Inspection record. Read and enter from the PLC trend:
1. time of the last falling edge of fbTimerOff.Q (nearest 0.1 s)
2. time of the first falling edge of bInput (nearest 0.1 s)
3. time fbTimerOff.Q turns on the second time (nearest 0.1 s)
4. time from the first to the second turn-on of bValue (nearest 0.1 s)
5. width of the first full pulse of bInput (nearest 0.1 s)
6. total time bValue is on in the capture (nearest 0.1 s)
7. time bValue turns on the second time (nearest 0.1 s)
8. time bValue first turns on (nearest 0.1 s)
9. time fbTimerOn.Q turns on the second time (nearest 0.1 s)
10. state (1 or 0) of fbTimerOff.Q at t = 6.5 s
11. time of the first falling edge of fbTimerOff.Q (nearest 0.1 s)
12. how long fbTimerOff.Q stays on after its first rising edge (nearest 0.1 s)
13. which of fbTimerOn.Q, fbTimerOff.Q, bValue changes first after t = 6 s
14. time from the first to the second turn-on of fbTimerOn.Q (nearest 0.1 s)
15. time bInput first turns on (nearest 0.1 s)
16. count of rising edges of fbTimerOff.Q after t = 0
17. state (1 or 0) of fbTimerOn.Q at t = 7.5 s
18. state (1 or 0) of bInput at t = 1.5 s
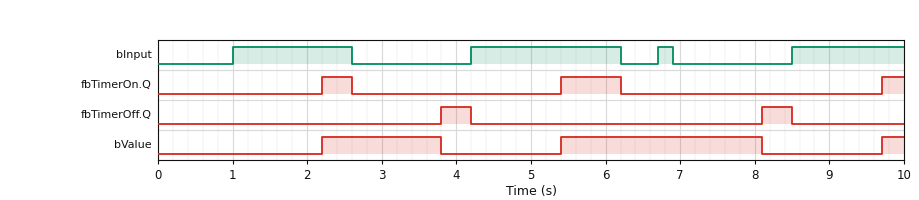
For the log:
8.5 s
2.6 s
8.1 s
3.2 s
1.6 s
4.6 s
5.4 s
2.2 s
5.4 s
0
4.2 s
0.4 s
fbTimerOn.Q
3.2 s
1.0 s
2
0
1
